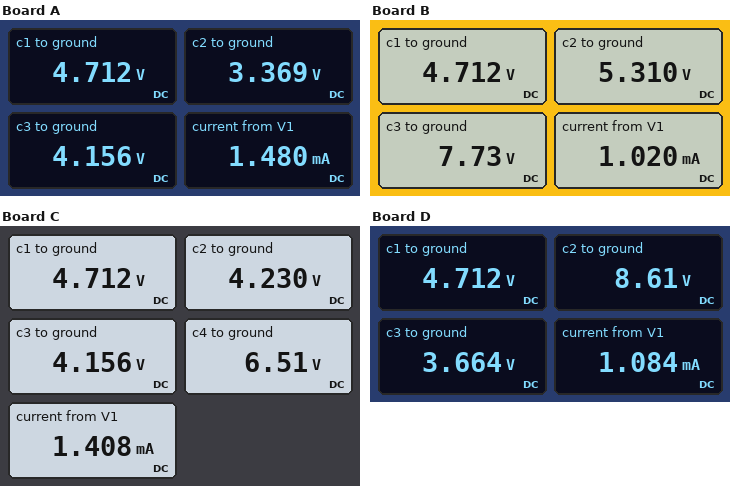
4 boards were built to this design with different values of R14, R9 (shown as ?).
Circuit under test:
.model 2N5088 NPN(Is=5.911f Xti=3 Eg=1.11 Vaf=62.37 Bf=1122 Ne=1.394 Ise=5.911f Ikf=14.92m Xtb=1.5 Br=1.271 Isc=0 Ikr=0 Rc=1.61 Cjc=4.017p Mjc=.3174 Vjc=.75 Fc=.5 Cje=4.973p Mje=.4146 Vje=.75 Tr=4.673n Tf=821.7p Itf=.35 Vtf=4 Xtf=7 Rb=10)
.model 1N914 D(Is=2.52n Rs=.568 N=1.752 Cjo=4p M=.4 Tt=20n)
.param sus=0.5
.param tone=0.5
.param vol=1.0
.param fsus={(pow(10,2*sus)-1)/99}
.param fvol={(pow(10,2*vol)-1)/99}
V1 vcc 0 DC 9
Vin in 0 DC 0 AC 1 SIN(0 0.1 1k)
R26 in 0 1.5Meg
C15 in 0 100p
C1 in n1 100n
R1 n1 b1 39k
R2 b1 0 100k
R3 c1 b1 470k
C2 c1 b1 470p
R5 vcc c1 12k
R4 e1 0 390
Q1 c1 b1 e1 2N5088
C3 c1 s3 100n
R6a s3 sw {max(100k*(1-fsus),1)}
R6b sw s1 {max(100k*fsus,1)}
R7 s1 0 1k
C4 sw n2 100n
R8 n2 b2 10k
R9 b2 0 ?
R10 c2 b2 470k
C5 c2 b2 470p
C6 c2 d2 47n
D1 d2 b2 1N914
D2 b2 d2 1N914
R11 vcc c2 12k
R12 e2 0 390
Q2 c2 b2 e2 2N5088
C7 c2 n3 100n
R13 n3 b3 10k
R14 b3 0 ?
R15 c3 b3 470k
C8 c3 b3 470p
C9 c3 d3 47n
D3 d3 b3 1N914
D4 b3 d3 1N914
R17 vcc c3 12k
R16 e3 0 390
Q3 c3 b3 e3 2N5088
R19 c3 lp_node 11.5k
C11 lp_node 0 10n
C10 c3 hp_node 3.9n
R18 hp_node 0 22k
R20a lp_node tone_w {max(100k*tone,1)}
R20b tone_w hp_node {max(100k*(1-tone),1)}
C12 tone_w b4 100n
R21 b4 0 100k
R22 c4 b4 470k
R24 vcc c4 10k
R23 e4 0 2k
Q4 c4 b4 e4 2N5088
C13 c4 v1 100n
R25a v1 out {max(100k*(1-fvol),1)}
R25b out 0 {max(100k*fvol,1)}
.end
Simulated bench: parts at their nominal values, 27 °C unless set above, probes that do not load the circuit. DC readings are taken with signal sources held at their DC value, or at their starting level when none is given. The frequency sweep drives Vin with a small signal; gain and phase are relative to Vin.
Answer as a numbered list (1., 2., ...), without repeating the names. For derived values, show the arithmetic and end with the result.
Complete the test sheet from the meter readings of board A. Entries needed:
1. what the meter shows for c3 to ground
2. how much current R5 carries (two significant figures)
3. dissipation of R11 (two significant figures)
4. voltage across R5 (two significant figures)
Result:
1. 4.156 V
2. (9 V - 4.712 V) / 12 kΩ = 360 µA
3. (9 V - 3.369 V)^2 / 12 kΩ = 2.6 mW
4. 9 V - 4.712 V = 4.3 V
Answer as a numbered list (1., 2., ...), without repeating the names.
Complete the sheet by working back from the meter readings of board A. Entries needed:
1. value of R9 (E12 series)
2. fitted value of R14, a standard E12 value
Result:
1. 180 kΩ
2. 120 kΩ
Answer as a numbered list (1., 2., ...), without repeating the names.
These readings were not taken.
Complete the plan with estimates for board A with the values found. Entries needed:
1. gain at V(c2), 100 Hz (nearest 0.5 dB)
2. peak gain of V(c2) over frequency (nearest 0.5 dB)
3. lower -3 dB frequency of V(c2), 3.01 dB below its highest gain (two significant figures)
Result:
1. 14.5 dB
2. 14.5 dB
3. 46 Hz
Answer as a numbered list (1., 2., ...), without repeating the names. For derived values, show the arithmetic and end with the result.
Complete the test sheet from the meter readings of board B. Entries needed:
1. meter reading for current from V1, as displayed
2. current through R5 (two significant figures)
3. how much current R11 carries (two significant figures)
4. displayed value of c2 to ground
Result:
1. 1.020 mA
2. (9 V - 4.712 V) / 12 kΩ = 360 µA
3. (9 V - 5.31 V) / 12 kΩ = 310 µA
4. 5.310 V
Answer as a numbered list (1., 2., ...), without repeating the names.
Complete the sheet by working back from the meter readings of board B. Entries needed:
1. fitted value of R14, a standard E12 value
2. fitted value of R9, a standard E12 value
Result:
1. 39 kΩ
2. 82 kΩ
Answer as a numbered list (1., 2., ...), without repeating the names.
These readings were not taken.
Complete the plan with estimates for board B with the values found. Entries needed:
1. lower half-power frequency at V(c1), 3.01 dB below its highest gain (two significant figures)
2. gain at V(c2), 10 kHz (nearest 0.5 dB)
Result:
1. 27 Hz
2. -18.5 dB
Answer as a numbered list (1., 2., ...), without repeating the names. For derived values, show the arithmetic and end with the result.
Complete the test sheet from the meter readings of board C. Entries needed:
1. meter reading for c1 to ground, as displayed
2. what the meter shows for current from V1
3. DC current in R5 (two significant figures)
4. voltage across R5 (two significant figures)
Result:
1. 4.712 V
2. 1.408 mA
3. (9 V - 4.712 V) / 12 kΩ = 360 µA
4. 9 V - 4.712 V = 4.3 V
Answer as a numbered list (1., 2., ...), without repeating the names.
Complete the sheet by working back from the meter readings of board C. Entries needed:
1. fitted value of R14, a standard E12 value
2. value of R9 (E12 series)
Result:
1. 120 kΩ
2. 120 kΩ
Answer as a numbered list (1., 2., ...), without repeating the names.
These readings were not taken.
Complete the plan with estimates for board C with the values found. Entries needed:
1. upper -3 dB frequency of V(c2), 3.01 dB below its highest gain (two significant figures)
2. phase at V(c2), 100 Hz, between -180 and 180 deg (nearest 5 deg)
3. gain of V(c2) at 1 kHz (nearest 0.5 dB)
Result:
1. 970 Hz
2. 35 deg
3. 11.0 dB
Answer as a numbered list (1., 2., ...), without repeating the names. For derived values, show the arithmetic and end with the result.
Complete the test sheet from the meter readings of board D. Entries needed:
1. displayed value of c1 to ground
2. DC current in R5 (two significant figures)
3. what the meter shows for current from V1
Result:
1. 4.712 V
2. (9 V - 4.712 V) / 12 kΩ = 360 µA
3. 1.084 mA
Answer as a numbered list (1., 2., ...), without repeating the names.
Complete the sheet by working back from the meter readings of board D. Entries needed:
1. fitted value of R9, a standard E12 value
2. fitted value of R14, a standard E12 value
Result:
1. 33 kΩ
2. 150 kΩ
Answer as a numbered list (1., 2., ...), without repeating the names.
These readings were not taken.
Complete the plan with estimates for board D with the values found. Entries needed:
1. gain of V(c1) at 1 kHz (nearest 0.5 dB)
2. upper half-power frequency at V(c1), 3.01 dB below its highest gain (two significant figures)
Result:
1. 14.0 dB
2. 1.3 kHz
